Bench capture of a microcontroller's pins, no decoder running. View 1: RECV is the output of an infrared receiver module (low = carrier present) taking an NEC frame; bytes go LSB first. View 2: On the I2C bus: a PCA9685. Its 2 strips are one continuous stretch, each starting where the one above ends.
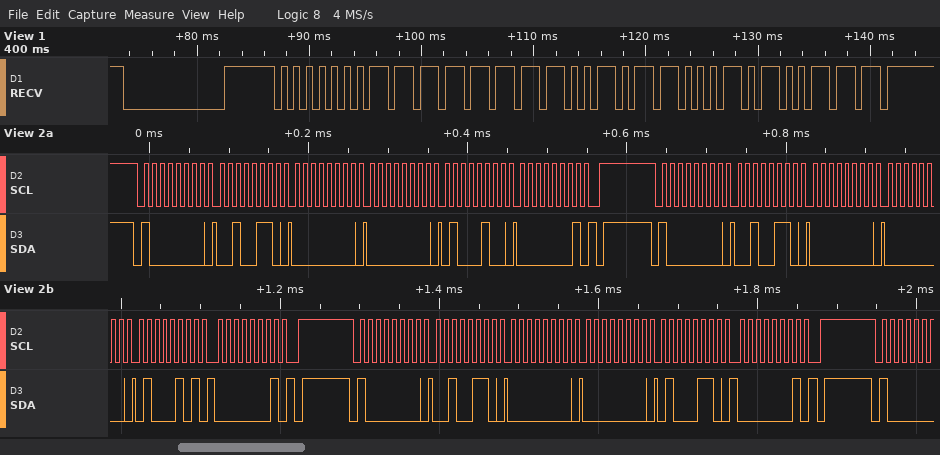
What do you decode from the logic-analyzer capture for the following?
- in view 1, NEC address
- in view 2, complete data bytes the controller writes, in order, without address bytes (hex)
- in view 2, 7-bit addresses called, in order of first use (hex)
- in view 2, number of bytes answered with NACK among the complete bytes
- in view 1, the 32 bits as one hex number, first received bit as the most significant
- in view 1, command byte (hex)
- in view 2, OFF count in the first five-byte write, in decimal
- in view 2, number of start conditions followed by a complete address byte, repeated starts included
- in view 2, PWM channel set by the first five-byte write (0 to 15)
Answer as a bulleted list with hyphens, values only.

- 0x80
- 26 00 00 44 01 26 00 00 45 01 26 00 00 46 01
- 0x40
- 0
- 0x01FE58A7
- 0x1A
- 324
- 3
- 8
